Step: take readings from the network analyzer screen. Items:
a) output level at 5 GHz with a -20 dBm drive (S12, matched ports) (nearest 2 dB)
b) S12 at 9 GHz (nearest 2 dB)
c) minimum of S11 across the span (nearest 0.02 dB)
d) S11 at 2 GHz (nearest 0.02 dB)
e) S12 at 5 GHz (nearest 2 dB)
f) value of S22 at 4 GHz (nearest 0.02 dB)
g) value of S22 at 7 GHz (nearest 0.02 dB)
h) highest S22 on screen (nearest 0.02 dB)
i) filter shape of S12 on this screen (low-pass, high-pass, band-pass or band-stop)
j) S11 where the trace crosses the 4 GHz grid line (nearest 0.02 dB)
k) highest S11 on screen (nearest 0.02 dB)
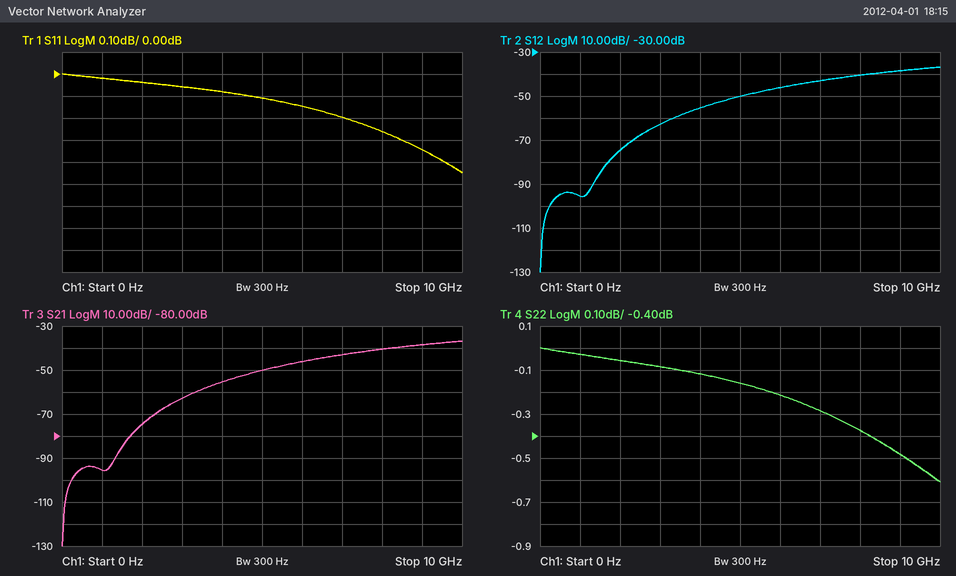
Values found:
-70 dBm
-38 dB
-0.44 dB
-0.04 dB
-50 dB
-0.12 dB
-0.28 dB
0.00 dB
high-pass
-0.08 dB
0.00 dB
